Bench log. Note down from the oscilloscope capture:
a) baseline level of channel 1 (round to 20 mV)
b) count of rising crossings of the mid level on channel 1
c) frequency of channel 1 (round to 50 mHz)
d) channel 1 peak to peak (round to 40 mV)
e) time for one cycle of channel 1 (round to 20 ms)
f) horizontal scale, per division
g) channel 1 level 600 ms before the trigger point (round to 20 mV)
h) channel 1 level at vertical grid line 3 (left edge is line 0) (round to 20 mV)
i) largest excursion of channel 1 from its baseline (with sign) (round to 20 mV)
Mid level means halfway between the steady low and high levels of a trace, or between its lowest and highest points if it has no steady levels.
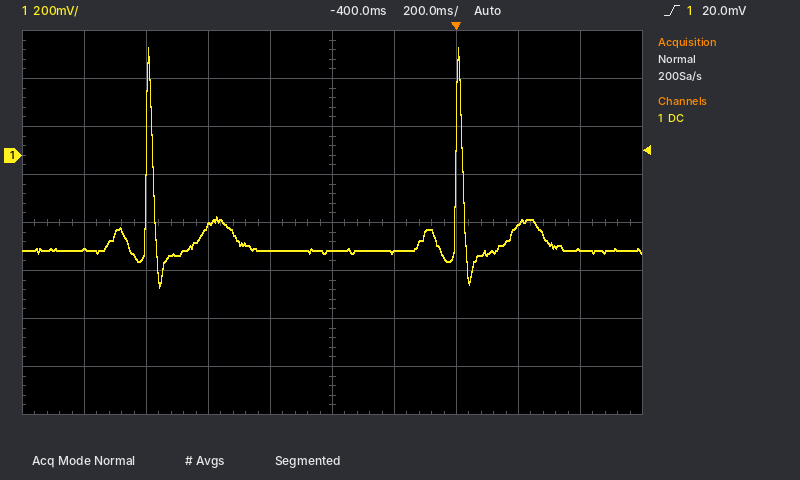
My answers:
-400 mV
2
1.00 Hz
1.00 V
1.00 s
200 ms
-400 mV
-300 mV
+840 mV
